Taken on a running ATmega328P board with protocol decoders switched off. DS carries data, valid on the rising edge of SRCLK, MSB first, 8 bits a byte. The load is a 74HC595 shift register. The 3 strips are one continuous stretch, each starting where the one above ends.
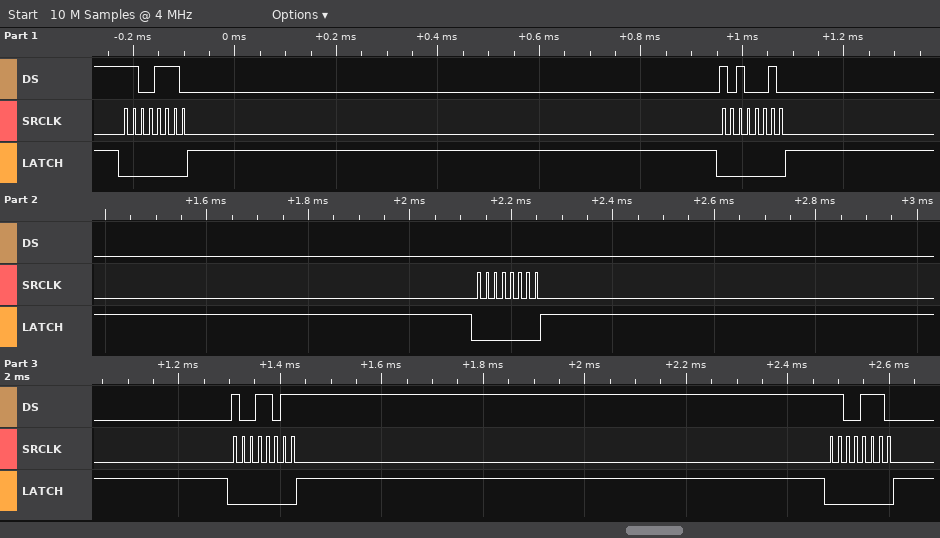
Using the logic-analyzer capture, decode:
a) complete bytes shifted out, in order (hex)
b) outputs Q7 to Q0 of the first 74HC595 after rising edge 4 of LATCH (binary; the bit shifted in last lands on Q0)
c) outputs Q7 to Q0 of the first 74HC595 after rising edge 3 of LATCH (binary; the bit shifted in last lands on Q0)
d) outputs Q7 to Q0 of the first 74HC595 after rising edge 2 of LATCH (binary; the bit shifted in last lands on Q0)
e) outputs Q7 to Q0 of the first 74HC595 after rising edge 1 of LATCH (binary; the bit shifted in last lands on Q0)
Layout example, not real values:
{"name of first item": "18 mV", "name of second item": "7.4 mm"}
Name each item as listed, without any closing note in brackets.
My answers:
{"complete bytes shifted out, in order": "0xCE 0xA2 0x00 0x9B 0xCE", "outputs Q7 to Q0 of the first 74HC595 after rising edge 4 of LATCH": "10011011", "outputs Q7 to Q0 of the first 74HC595 after rising edge 3 of LATCH": "00000000", "outputs Q7 to Q0 of the first 74HC595 after rising edge 2 of LATCH": "10100010", "outputs Q7 to Q0 of the first 74HC595 after rising edge 1 of LATCH": "11001110"}
